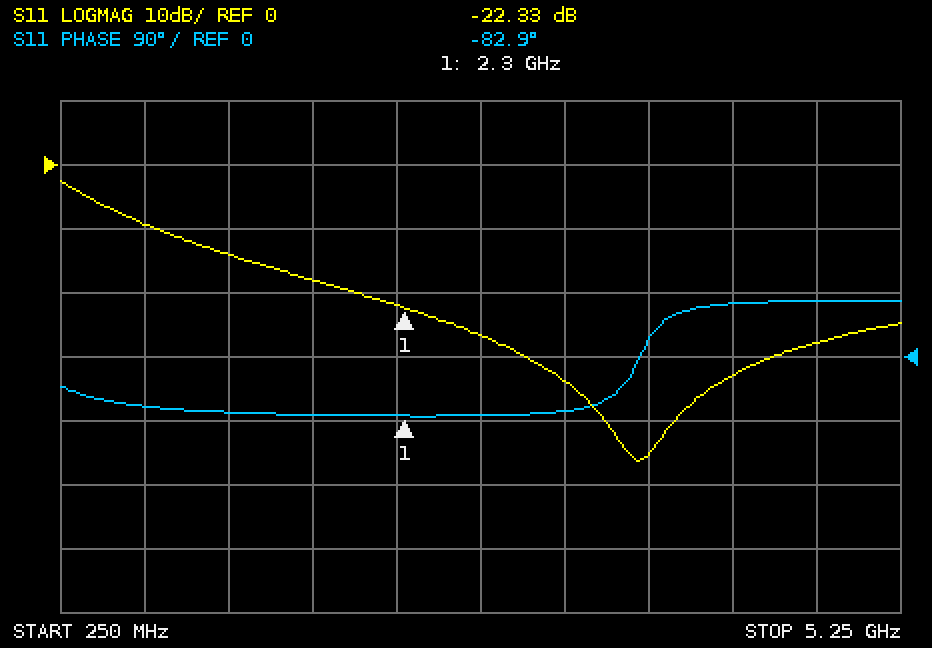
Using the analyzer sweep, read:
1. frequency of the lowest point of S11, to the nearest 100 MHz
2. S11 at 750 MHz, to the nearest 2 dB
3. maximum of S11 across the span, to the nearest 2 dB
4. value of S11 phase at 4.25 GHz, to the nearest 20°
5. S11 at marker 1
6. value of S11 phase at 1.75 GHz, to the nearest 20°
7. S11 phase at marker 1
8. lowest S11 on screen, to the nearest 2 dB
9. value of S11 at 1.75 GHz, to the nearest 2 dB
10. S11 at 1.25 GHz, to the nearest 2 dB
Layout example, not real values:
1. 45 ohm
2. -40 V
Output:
1. 3.7 GHz
2. -10 dB
3. -2 dB
4. 80°
5. -22.33 dB
6. -80°
7. -82.9°
8. -46 dB
9. -18 dB
10. -14 dB
